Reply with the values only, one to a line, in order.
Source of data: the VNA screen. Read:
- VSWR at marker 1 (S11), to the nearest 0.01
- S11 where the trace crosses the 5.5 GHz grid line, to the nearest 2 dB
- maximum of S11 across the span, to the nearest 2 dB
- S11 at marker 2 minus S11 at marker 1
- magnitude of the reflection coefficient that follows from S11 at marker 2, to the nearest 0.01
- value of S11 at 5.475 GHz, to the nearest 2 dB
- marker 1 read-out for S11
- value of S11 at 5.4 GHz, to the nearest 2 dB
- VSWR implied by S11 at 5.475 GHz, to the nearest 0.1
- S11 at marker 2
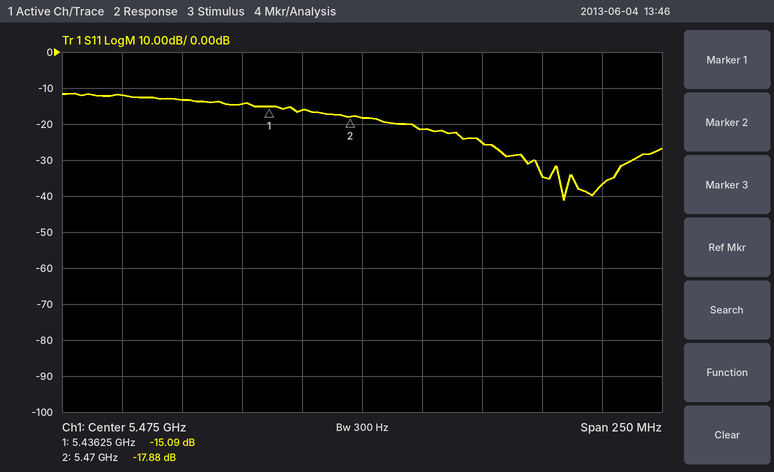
1.43
-22 dB
-12 dB
-2.79 dB
0.13
-18 dB
-15.09 dB
-14 dB
1.3
-17.88 dB
